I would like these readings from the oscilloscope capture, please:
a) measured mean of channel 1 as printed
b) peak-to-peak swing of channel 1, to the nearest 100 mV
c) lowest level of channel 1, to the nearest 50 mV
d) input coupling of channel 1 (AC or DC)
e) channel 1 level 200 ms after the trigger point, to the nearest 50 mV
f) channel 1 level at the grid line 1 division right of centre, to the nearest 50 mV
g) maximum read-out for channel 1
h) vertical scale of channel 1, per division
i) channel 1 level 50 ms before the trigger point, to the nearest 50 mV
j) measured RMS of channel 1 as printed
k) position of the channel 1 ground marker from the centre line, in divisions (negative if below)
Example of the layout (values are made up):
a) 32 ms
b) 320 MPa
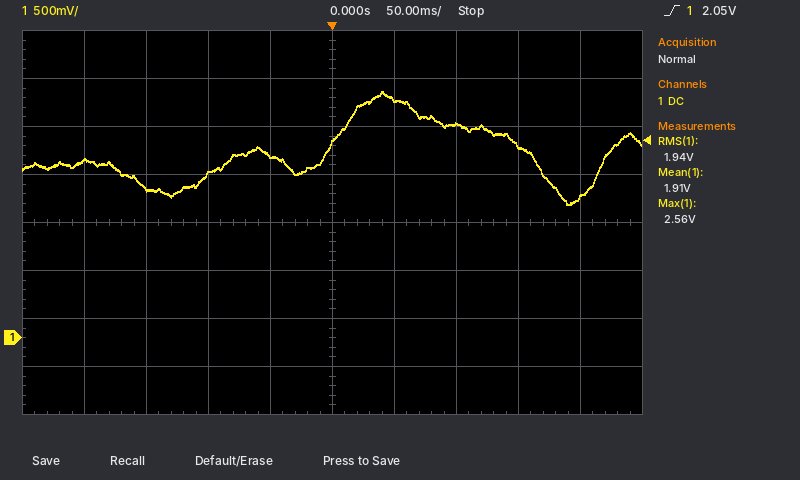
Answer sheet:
a) 1.91 V
b) 1.20 V
c) 1.40 V
d) DC
e) 1.45 V
f) 2.50 V
g) 2.56 V
h) 500 mV
i) 1.90 V
j) 1.94 V
k) -2.4 div
